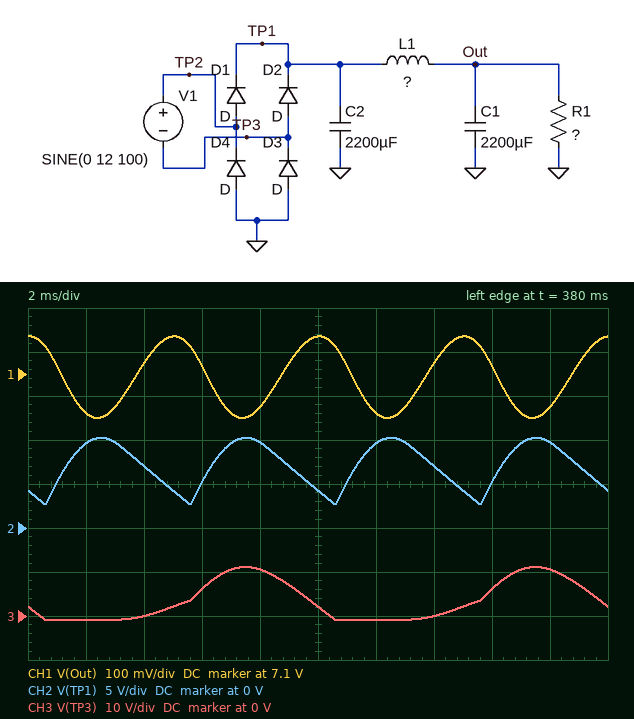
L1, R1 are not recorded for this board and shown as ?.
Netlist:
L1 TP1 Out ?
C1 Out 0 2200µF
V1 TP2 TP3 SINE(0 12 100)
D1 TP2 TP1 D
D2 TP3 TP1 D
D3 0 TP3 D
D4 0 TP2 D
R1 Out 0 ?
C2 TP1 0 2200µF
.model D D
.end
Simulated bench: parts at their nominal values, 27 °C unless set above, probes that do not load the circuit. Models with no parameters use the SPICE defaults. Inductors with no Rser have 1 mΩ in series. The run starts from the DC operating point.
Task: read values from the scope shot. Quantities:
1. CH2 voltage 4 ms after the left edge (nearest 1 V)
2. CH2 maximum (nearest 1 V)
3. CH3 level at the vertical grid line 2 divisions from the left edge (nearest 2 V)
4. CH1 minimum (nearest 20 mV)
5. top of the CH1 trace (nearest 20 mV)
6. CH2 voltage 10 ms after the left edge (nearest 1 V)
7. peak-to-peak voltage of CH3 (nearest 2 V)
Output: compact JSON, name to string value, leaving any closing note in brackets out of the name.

{"CH2 voltage 4 ms after the left edge": "7 V", "CH2 maximum": "10 V", "CH3 level at the vertical grid line 2 divisions from the left edge": "0 V", "CH1 minimum": "7.00 V", "top of the CH1 trace": "7.18 V", "CH2 voltage 10 ms after the left edge": "4 V", "peak-to-peak voltage of CH3": "12 V"}
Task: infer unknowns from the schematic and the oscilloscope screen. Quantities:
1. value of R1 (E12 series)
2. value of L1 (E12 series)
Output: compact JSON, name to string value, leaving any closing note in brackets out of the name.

{"value of R1": "1.2 Ω", "value of L1": "10 mH"}
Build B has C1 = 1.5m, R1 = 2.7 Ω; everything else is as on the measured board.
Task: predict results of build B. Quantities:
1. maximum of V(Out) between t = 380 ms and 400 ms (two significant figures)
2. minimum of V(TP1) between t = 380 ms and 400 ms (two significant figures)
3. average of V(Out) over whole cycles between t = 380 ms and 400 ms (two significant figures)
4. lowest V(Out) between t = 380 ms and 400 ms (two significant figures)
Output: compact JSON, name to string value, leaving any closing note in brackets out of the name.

{"maximum of V(Out) between t = 380 ms and 400 ms": "8.3 V", "minimum of V(TP1) between t = 380 ms and 400 ms": "5.6 V", "average of V(Out) over whole cycles between t = 380 ms and 400 ms": "8.2 V", "lowest V(Out) between t = 380 ms and 400 ms": "8.1 V"}
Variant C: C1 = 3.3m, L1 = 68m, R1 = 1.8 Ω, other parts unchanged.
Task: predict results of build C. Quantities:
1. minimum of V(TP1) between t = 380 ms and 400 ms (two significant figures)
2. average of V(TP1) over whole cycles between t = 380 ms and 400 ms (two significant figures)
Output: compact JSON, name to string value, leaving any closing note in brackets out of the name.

{"minimum of V(TP1) between t = 380 ms and 400 ms": "4.3 V", "average of V(TP1) over whole cycles between t = 380 ms and 400 ms": "7.7 V"}
